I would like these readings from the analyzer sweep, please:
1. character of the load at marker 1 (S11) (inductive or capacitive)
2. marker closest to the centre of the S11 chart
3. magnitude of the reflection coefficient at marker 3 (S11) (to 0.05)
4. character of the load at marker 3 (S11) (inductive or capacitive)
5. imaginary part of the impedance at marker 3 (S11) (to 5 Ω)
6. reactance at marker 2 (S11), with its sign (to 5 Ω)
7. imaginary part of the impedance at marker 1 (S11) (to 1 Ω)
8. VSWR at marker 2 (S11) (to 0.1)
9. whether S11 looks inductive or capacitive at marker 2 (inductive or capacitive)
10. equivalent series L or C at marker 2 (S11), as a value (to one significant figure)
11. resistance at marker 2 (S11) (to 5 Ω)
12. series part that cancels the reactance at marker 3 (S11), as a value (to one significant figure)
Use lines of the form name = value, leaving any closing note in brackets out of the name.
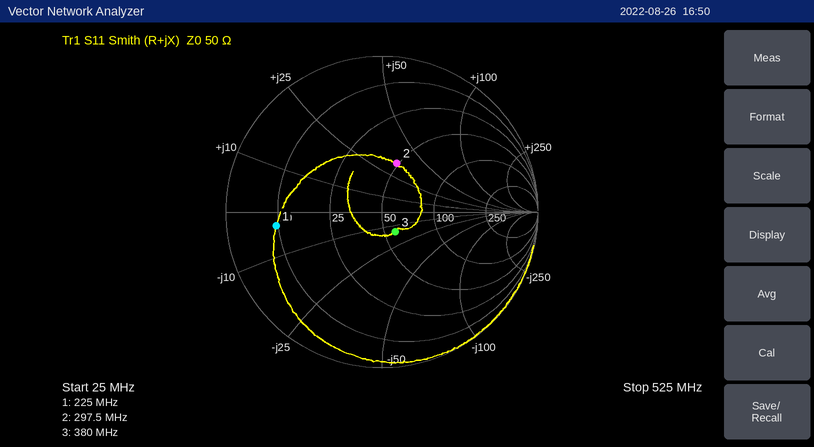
character of the load at marker 1 (S11) = capacitive
marker closest to the centre of the S11 chart = marker 3
magnitude of the reflection coefficient at marker 3 (S11) = 0.15
character of the load at marker 3 (S11) = capacitive
imaginary part of the impedance at marker 3 (S11) = -15 Ω
reactance at marker 2 (S11), with its sign = +35 Ω
imaginary part of the impedance at marker 1 (S11) = -3 Ω
VSWR at marker 2 (S11) = 2.0
whether S11 looks inductive or capacitive at marker 2 = inductive
equivalent series L or C at marker 2 (S11), as a value = 20 nH
resistance at marker 2 (S11) = 50 Ω
series part that cancels the reactance at marker 3 (S11), as a value = 6 nH
